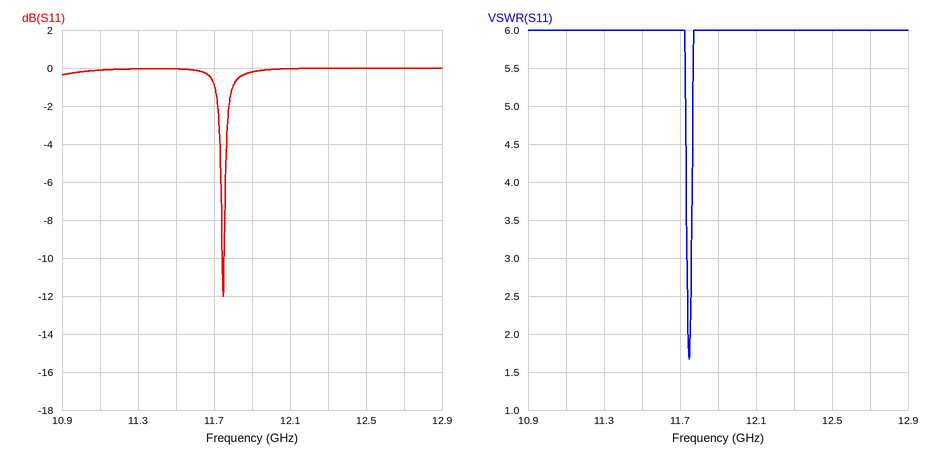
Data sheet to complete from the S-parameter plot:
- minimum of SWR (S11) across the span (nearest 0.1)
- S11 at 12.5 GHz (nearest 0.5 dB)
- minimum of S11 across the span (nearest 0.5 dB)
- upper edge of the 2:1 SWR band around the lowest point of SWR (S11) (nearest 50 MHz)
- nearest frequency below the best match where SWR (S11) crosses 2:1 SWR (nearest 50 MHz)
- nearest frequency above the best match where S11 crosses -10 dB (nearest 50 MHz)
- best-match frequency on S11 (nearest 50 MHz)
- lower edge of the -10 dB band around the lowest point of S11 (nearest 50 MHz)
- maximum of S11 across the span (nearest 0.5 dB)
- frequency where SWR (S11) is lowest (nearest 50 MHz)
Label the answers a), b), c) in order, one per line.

a) 1.7
b) 0.0 dB
c) -12.0 dB
d) 11.75 GHz
e) 11.75 GHz
f) 11.75 GHz
g) 11.75 GHz
h) 11.75 GHz
i) 0.0 dB
j) 11.75 GHz
